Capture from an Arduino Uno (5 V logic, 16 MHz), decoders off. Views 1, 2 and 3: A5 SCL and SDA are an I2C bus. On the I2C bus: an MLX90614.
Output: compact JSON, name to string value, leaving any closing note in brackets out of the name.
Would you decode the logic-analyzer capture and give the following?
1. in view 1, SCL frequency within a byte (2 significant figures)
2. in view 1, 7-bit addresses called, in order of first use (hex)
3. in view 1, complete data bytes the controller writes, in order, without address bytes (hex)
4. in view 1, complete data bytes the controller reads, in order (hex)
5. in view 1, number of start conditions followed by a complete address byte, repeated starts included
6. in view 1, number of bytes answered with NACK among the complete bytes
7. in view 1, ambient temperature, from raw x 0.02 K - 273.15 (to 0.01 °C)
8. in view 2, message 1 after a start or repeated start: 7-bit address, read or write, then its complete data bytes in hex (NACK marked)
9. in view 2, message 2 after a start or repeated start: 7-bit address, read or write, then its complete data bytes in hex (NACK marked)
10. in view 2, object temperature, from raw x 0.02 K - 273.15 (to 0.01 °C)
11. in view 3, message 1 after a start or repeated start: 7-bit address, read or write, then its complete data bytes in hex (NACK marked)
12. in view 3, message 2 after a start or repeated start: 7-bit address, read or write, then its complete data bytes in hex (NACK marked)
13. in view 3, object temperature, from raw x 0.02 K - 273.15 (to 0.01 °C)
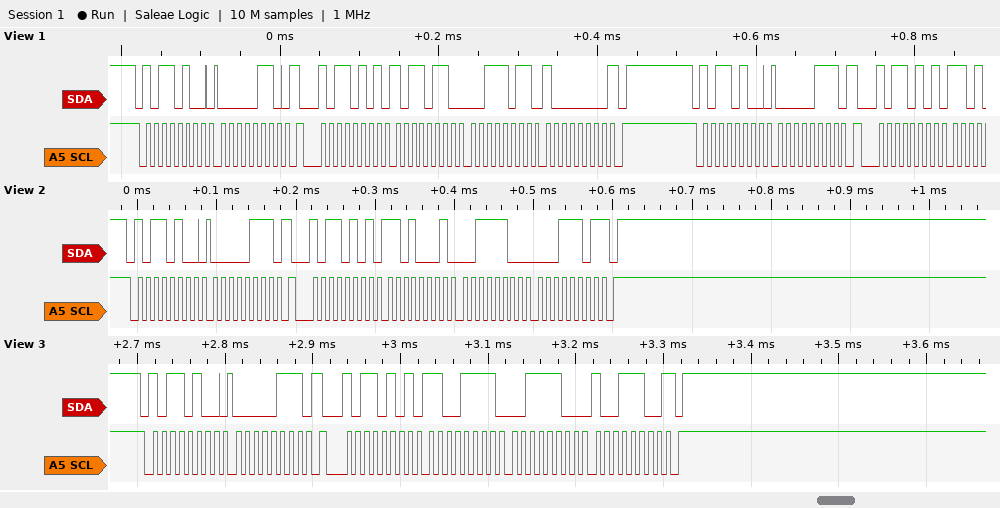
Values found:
{"in view 1, SCL frequency within a byte": "100 kHz", "in view 1, 7-bit addresses called, in order of first use": "0x5A", "in view 1, complete data bytes the controller writes, in order, without address bytes": "06 07", "in view 1, complete data bytes the controller reads, in order": "B6 3B 80", "in view 1, number of start conditions followed by a complete address byte, repeated starts included": "4", "in view 1, number of bytes answered with NACK among the complete bytes": "1", "in view 1, ambient temperature, from raw x 0.02 K - 273.15": "32.57 °C", "in view 2, message 1 after a start or repeated start: 7-bit address, read or write, then its complete data bytes in hex": "0x5A write: 07", "in view 2, message 2 after a start or repeated start: 7-bit address, read or write, then its complete data bytes in hex": "0x5A read: D1 3C 1D NACK", "in view 2, object temperature, from raw x 0.02 K - 273.15": "38.23 °C", "in view 3, message 1 after a start or repeated start: 7-bit address, read or write, then its complete data bytes in hex": "0x5A write: 07", "in view 3, message 2 after a start or repeated start: 7-bit address, read or write, then its complete data bytes in hex": "0x5A read: CF 3C 9C NACK", "in view 3, object temperature, from raw x 0.02 K - 273.15": "38.19 °C"}
